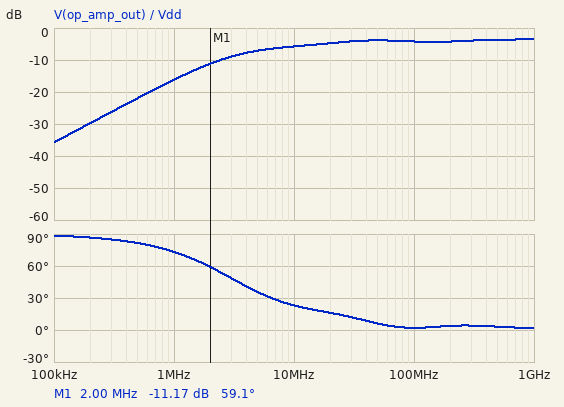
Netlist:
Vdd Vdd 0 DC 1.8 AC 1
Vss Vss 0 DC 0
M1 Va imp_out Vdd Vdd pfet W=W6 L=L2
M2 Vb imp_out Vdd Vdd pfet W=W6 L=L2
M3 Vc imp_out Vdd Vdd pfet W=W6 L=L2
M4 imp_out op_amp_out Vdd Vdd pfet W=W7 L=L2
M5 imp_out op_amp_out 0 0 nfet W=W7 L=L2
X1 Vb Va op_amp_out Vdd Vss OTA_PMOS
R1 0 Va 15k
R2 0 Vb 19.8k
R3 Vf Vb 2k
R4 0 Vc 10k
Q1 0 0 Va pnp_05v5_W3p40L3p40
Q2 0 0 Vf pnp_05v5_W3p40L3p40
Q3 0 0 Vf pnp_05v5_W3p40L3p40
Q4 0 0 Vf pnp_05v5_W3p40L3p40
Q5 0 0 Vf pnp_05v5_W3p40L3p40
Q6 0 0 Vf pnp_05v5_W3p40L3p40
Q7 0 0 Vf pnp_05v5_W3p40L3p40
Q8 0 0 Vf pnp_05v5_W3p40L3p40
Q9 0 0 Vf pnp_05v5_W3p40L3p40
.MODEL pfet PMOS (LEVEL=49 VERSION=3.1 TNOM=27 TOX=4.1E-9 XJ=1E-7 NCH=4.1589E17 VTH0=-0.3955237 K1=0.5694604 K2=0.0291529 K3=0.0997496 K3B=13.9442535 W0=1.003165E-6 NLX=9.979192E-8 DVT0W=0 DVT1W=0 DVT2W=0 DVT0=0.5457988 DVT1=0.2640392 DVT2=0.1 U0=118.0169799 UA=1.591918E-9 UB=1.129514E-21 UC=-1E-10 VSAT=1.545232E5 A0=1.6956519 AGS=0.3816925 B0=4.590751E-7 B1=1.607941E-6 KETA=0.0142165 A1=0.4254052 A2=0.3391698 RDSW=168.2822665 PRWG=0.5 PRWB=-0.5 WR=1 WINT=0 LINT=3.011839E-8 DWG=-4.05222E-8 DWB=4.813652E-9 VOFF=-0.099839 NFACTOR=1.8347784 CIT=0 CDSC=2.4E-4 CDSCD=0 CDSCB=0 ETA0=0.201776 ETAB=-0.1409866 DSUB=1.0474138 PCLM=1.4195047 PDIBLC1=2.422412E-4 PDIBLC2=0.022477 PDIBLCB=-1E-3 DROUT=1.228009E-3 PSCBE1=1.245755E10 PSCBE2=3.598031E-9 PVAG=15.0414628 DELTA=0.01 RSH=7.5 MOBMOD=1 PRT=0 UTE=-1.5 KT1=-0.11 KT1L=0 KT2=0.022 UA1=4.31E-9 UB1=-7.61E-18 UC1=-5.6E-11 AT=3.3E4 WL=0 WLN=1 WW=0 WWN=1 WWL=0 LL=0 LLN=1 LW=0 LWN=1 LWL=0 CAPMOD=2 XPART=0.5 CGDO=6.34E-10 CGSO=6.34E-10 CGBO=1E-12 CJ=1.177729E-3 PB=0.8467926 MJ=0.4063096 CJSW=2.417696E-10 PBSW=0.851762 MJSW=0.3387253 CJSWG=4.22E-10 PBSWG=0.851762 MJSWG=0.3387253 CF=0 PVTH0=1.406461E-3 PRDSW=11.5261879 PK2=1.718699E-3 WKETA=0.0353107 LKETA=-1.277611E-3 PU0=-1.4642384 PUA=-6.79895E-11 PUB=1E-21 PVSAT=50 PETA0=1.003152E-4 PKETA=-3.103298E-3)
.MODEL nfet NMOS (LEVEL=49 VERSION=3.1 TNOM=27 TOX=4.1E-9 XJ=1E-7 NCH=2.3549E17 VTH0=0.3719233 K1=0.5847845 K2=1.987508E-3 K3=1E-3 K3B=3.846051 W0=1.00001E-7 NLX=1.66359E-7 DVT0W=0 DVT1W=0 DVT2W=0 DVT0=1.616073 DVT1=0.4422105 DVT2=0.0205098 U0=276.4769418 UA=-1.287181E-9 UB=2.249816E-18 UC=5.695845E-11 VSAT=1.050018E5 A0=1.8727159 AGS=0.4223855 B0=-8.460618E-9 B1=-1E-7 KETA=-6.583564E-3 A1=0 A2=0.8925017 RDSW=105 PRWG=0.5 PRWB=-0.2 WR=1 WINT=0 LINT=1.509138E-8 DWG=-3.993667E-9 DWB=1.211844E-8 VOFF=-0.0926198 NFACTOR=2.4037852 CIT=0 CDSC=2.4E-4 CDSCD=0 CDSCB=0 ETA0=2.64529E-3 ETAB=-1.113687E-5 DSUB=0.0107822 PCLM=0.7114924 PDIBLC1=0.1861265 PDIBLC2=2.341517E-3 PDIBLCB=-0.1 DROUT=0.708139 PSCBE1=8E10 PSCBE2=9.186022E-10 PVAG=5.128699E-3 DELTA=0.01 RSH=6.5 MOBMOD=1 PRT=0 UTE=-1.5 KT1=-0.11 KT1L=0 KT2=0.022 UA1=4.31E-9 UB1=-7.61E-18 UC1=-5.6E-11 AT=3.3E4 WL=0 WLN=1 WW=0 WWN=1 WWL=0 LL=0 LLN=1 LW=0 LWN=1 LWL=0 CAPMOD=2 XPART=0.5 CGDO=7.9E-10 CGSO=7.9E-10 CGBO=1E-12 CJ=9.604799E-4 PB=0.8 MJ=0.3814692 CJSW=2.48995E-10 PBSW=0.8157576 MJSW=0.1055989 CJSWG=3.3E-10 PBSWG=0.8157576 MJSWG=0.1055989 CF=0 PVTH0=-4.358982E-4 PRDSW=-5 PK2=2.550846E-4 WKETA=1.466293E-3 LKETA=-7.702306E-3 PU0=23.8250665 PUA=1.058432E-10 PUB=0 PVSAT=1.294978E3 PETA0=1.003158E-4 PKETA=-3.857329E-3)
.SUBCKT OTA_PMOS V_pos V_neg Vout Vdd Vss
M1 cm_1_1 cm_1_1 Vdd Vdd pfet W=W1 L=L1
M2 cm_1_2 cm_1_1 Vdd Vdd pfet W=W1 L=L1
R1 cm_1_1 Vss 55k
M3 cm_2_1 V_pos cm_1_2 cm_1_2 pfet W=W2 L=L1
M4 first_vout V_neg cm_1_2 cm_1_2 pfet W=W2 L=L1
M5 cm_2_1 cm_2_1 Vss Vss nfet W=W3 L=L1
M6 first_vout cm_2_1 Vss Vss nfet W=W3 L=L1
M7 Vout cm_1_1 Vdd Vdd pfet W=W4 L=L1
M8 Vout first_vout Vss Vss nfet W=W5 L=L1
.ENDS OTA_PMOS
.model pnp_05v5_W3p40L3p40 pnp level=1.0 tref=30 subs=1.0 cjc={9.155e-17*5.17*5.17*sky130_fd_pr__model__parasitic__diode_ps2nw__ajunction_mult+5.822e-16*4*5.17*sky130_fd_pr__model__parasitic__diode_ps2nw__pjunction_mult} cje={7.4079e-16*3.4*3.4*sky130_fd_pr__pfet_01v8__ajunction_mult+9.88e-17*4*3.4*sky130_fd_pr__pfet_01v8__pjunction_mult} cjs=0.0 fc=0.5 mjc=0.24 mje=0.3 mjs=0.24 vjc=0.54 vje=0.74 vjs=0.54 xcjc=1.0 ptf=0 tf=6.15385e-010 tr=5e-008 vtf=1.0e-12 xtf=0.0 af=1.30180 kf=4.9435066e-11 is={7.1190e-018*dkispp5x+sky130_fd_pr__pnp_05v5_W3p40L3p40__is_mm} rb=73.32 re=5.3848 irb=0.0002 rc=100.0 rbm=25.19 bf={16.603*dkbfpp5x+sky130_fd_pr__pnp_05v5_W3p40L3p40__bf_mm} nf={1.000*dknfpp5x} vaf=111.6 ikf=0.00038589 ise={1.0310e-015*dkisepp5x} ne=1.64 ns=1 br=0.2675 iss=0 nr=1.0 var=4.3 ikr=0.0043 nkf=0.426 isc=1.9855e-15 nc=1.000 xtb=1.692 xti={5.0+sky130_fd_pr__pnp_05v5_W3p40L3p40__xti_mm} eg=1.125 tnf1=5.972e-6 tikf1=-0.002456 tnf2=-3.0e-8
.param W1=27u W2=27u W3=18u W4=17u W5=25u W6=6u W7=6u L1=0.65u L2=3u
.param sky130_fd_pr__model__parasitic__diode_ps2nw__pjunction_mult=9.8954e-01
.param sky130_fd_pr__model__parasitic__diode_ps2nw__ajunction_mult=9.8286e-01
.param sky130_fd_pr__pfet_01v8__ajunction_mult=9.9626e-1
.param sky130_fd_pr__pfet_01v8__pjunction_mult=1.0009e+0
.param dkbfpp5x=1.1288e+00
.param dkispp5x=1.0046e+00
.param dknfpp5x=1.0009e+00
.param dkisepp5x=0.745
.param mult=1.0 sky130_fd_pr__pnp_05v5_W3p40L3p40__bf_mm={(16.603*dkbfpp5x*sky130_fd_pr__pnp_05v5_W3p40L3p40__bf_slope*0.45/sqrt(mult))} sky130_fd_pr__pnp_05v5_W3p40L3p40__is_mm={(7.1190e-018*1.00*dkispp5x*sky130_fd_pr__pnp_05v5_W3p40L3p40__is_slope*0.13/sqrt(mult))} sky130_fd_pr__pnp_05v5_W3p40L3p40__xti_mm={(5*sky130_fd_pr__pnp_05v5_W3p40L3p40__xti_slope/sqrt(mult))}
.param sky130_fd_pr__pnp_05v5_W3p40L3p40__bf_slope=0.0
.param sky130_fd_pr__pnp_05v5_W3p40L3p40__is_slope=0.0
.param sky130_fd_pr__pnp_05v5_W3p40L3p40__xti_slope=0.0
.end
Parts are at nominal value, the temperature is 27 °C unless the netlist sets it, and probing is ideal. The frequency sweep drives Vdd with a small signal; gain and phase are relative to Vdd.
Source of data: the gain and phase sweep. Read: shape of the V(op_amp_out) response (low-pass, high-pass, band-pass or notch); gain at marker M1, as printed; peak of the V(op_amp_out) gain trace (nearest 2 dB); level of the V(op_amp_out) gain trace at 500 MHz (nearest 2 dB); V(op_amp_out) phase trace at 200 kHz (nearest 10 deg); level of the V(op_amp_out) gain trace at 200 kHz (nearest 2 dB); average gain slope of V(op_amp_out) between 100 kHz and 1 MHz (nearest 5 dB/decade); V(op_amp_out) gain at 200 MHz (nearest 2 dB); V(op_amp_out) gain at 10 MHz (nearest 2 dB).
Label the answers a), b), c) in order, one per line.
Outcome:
a) high-pass
b) -11.17 dB
c) -4 dB
d) -4 dB
e) 90 deg
f) -30 dB
g) 20 dB/decade
h) -4 dB
i) -6 dB
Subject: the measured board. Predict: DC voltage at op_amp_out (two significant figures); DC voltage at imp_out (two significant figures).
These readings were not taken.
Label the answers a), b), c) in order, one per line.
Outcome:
a) 200 mV
b) 1.8 V
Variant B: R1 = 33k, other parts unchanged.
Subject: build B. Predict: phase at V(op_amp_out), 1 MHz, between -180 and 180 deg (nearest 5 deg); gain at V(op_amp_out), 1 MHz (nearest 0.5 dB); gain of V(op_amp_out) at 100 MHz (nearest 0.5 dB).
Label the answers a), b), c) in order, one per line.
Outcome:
a) 70 deg
b) -13.0 dB
c) -5.0 dB
